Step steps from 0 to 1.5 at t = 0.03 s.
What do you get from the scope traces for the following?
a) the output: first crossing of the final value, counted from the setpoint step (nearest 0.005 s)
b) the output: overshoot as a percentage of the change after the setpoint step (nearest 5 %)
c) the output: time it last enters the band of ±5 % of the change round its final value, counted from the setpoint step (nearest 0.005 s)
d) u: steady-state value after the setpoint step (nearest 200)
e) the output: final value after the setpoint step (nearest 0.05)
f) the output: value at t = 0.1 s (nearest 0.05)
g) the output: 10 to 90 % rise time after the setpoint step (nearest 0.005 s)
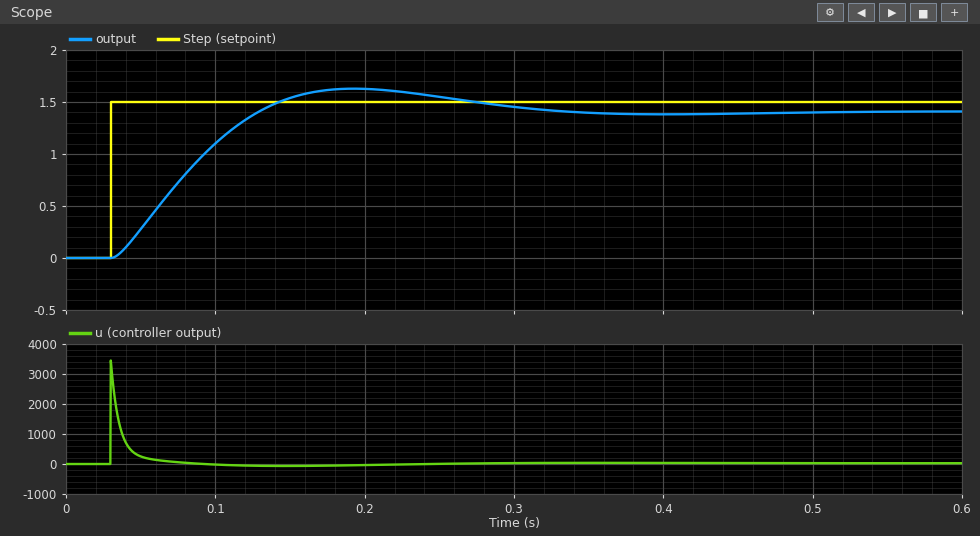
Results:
0.100 s
15 %
0.255 s
0
1.40
1.10
0.070 s
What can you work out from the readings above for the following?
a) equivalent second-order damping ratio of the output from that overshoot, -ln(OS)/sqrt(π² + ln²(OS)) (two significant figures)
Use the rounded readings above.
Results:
0.52
